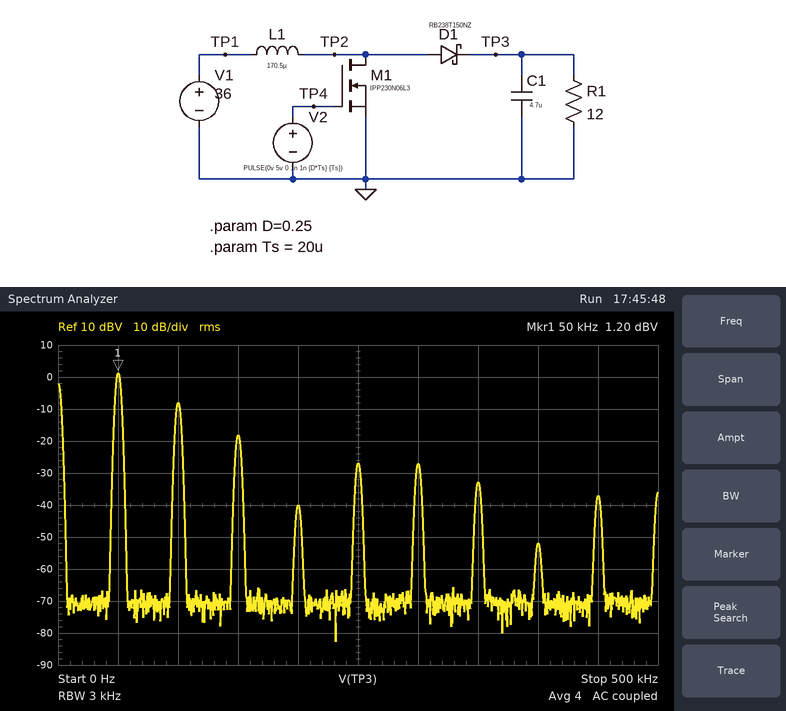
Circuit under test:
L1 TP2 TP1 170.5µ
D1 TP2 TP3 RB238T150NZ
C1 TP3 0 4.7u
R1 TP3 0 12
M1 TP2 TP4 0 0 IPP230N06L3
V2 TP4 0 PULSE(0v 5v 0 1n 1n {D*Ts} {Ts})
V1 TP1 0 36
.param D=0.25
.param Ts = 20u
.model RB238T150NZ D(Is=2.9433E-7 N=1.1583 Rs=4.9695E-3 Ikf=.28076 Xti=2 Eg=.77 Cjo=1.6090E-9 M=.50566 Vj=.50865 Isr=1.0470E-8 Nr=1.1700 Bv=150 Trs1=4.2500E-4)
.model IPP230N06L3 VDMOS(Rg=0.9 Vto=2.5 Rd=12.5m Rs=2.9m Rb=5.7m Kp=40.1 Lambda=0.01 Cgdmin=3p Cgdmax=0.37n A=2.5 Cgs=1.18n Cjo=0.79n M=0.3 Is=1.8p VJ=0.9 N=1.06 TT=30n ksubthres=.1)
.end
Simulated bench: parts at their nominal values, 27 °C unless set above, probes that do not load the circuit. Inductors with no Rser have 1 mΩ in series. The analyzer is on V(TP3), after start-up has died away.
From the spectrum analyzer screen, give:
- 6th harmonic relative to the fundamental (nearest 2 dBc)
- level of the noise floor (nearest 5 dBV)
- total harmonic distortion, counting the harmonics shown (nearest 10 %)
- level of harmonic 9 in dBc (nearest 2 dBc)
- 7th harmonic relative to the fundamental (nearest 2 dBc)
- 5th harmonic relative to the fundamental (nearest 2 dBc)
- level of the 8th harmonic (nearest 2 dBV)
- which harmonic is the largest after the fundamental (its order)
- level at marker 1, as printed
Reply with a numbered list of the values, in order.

1. -28 dBc
2. -70 dBV
3. 40 %
4. -38 dBc
5. -34 dBc
6. -28 dBc
7. -52 dBV
8. 2
9. 1.20 dBV
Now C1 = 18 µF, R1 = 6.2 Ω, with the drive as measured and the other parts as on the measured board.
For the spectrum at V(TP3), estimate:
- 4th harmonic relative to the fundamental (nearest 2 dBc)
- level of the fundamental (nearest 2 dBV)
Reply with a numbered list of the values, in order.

1. -46 dBc
2. -4 dBV
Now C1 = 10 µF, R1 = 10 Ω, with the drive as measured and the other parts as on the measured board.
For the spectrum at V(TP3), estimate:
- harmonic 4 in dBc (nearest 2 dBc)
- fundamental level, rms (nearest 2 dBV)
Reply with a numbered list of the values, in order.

1. -42 dBc
2. -4 dBV
